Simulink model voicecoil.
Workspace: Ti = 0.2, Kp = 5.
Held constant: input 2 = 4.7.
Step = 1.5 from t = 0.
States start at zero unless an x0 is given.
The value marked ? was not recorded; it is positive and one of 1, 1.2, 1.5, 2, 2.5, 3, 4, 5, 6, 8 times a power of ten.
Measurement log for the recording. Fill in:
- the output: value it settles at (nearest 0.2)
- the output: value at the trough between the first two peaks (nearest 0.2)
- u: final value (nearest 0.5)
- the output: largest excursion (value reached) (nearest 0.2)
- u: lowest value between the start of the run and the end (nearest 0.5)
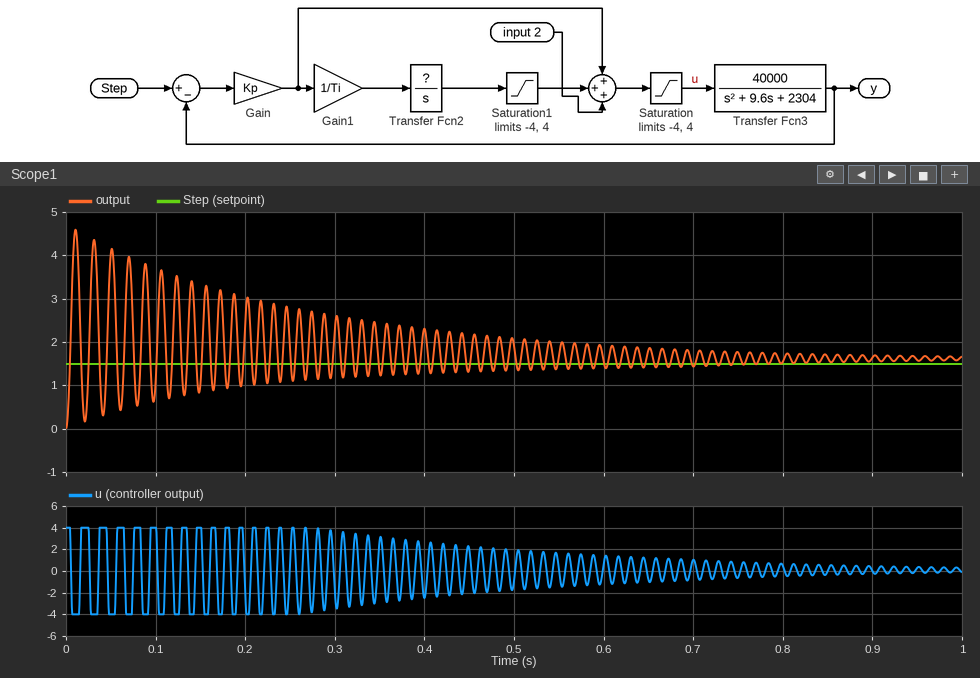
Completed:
1.6
0.2
0.0
4.6
-4.0
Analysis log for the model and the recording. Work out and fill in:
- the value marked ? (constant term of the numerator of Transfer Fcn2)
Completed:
0.6
